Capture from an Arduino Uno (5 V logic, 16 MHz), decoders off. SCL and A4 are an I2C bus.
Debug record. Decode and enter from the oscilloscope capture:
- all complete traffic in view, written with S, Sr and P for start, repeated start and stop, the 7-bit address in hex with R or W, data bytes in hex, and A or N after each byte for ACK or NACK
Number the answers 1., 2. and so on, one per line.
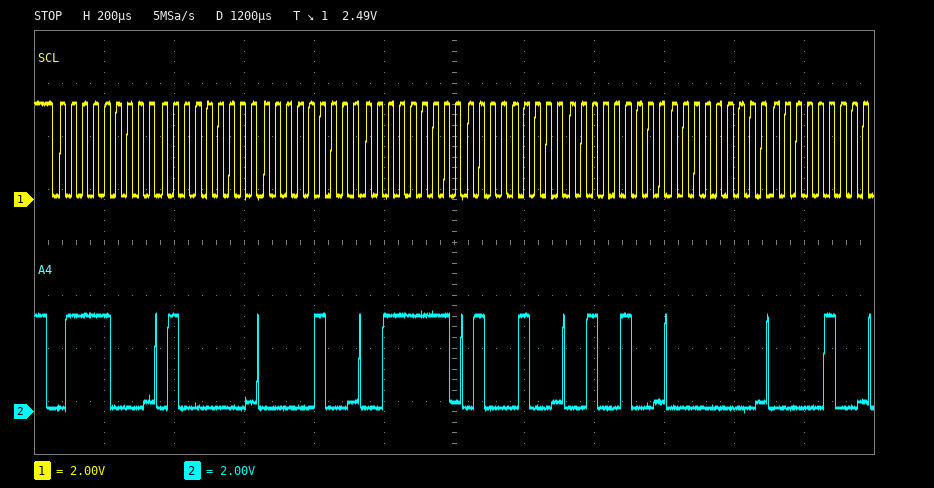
1. S 3CW A 40 A 04 A 3F A 44 A 24 A 00 A 04 A
